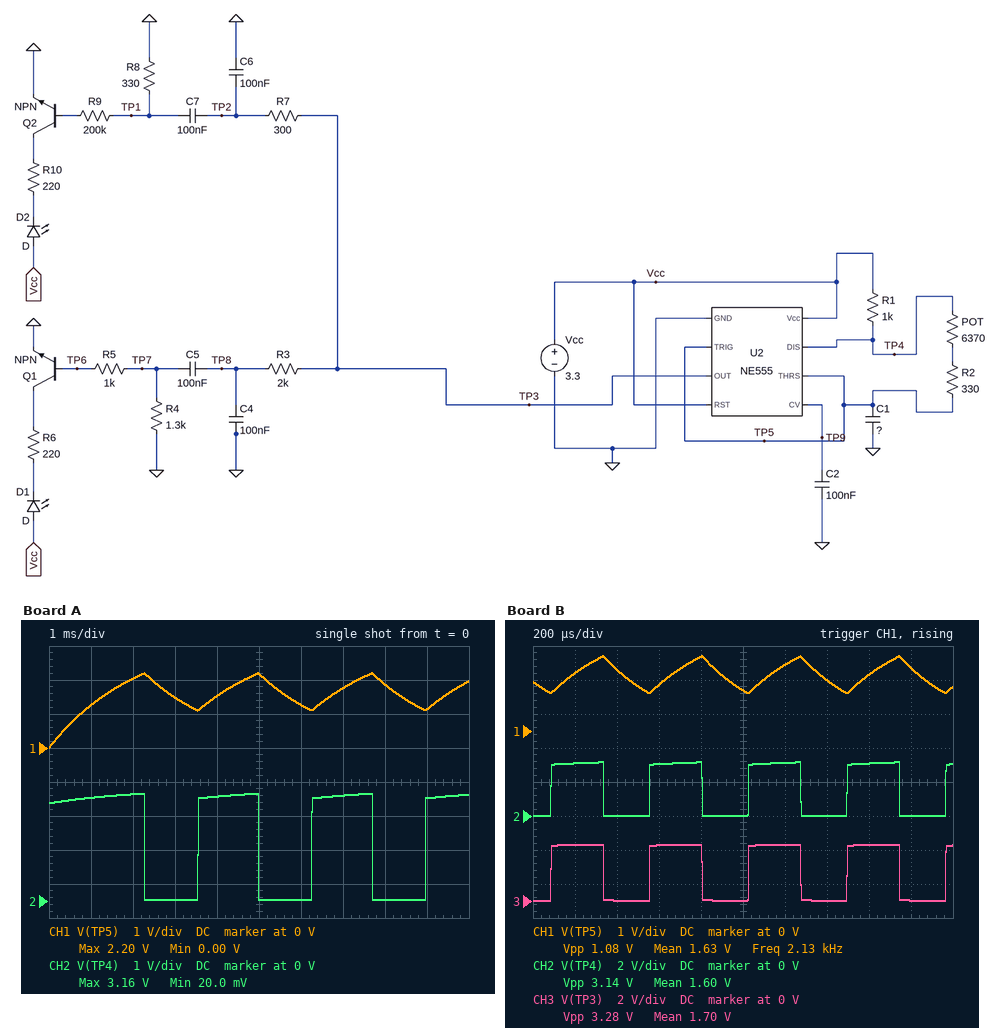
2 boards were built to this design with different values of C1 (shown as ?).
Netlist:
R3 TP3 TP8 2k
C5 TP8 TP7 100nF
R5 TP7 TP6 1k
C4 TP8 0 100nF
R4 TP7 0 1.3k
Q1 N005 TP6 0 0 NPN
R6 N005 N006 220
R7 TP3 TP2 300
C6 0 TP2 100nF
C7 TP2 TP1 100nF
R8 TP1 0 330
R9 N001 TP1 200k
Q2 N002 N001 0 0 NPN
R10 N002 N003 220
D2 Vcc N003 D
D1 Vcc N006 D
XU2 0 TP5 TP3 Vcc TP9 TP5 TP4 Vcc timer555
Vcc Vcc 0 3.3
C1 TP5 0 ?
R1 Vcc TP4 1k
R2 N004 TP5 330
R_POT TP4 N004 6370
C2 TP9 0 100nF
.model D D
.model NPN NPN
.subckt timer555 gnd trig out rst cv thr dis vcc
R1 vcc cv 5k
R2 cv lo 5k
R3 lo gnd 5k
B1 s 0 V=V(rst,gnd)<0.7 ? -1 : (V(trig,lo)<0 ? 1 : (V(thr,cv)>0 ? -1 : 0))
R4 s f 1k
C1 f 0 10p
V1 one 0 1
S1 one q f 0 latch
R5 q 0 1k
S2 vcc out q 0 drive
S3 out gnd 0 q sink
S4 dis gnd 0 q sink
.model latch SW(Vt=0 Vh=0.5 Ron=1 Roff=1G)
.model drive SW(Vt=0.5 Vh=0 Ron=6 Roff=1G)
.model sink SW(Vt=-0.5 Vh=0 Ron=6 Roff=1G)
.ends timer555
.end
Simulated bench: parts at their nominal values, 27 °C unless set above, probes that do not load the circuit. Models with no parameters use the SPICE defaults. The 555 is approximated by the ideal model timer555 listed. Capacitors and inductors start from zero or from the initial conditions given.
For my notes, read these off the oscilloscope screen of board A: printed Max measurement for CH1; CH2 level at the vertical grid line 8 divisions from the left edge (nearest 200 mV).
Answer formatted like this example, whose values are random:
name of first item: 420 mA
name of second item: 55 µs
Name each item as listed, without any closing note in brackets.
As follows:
printed Max measurement for CH1: 2.20 V
CH2 level at the vertical grid line 8 divisions from the left edge: 0 V
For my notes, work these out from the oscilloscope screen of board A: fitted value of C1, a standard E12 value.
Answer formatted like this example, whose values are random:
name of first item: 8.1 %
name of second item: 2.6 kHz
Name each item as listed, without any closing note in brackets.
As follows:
fitted value of C1, a standard E12 value: 270 nF
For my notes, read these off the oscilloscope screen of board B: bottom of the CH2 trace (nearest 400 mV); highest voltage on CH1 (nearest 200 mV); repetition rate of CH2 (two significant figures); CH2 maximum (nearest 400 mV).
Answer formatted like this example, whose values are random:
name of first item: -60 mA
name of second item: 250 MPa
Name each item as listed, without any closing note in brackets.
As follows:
bottom of the CH2 trace: 0 V
highest voltage on CH1: 2.2 V
repetition rate of CH2: 2.1 kHz
CH2 maximum: 3.2 V
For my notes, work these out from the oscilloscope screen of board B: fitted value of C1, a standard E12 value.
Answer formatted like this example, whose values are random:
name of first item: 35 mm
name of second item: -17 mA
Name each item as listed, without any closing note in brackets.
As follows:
fitted value of C1, a standard E12 value: 47 nF
